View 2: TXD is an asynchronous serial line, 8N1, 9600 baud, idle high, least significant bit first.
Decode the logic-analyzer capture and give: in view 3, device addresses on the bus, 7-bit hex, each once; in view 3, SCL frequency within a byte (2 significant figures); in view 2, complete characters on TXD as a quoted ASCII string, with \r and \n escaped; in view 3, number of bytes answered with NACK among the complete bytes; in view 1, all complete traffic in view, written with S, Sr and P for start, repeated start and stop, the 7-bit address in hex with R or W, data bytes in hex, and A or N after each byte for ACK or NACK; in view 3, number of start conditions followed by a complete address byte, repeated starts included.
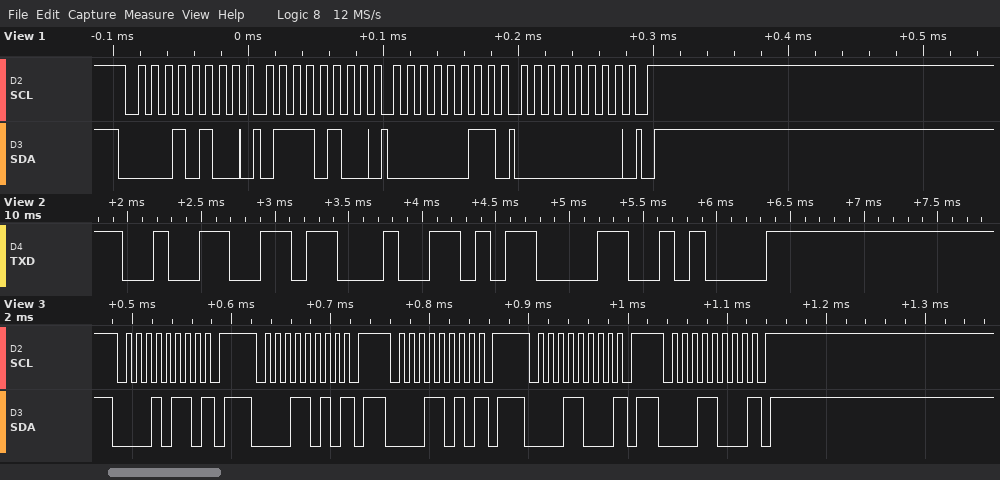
0x0B 0x0D 0x0C
100 kHz
"2#\r\n"
5
S 0AW A 74 A 03 A 00 A P
5
